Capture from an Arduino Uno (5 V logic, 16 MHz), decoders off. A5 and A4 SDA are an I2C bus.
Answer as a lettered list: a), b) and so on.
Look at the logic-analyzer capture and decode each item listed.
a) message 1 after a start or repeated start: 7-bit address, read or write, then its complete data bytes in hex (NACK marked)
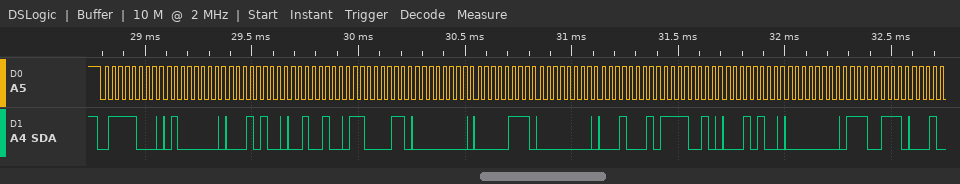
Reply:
a) 0x3C write: 40 14 24 C3 00 07 00 11 F2 14 00 E7
